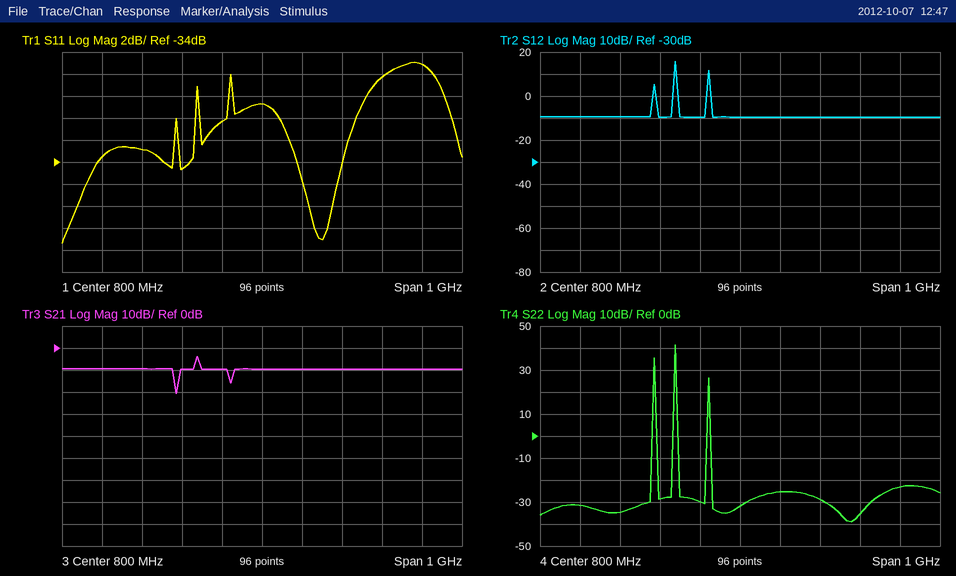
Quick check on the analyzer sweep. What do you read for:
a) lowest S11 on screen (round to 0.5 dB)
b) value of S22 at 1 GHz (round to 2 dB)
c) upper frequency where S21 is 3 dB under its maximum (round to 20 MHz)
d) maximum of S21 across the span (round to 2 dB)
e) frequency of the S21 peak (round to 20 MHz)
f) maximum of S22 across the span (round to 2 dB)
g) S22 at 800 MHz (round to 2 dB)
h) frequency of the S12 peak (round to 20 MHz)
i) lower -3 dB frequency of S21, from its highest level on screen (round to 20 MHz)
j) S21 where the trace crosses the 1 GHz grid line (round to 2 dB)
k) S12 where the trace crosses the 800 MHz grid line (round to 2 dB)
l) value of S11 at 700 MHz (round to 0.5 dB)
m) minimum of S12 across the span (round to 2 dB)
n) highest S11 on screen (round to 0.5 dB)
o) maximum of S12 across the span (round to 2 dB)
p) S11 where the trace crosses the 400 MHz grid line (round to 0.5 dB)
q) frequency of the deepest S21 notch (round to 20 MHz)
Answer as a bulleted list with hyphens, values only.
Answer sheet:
- -41.5 dB
- -28 dB
- 640 MHz
- -4 dB
- 640 MHz
- 42 dB
- -32 dB
- 640 MHz
- 640 MHz
- -10 dB
- -10 dB
- -30.5 dB
- -10 dB
- -25.0 dB
- 16 dB
- -33.5 dB
- 580 MHz
